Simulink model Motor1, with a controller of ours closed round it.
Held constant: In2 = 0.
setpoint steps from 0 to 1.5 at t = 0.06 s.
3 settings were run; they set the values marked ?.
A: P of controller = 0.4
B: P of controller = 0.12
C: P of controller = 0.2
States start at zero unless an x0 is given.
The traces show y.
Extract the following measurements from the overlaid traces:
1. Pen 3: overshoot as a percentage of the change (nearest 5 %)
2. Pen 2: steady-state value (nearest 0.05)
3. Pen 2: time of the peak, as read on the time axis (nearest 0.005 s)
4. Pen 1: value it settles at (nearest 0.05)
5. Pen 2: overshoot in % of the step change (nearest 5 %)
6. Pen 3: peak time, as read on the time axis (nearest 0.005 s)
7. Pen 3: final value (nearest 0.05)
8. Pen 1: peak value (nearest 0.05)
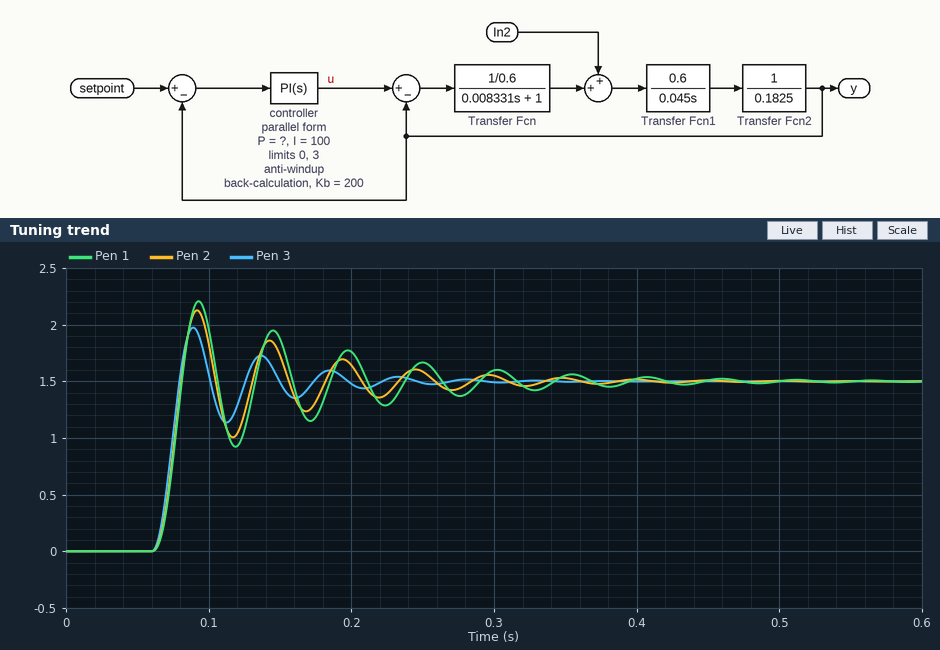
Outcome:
30 %
1.50
0.090 s
1.50
40 %
0.090 s
1.50
2.20
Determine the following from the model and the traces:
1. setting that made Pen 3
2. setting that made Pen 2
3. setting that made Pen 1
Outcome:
A
C
B
